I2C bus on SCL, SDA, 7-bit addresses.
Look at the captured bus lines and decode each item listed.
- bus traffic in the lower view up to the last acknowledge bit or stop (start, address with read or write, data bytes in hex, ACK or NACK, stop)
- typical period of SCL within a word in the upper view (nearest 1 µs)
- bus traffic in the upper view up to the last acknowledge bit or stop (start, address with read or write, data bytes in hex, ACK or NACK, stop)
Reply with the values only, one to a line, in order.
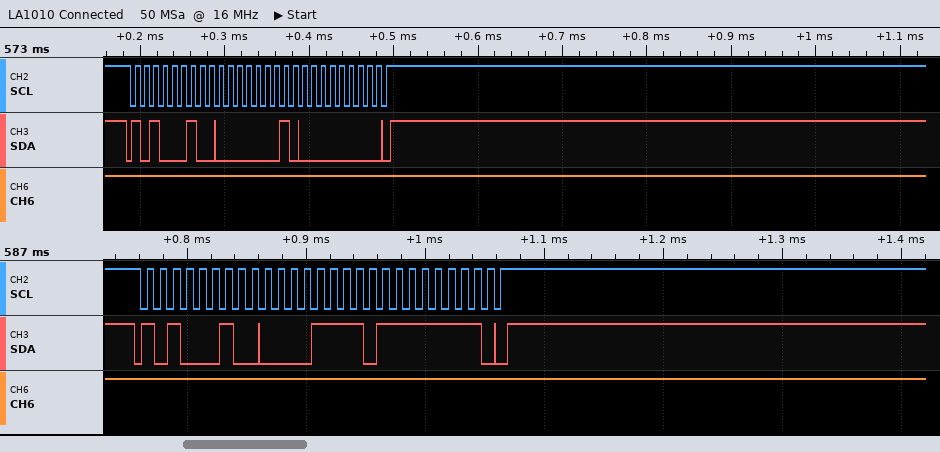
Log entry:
start, address 51 write ACK, 0F ACK, FF ACK, stop
11 µs
start, address 51 write ACK, 01 ACK, 00 ACK, stop
